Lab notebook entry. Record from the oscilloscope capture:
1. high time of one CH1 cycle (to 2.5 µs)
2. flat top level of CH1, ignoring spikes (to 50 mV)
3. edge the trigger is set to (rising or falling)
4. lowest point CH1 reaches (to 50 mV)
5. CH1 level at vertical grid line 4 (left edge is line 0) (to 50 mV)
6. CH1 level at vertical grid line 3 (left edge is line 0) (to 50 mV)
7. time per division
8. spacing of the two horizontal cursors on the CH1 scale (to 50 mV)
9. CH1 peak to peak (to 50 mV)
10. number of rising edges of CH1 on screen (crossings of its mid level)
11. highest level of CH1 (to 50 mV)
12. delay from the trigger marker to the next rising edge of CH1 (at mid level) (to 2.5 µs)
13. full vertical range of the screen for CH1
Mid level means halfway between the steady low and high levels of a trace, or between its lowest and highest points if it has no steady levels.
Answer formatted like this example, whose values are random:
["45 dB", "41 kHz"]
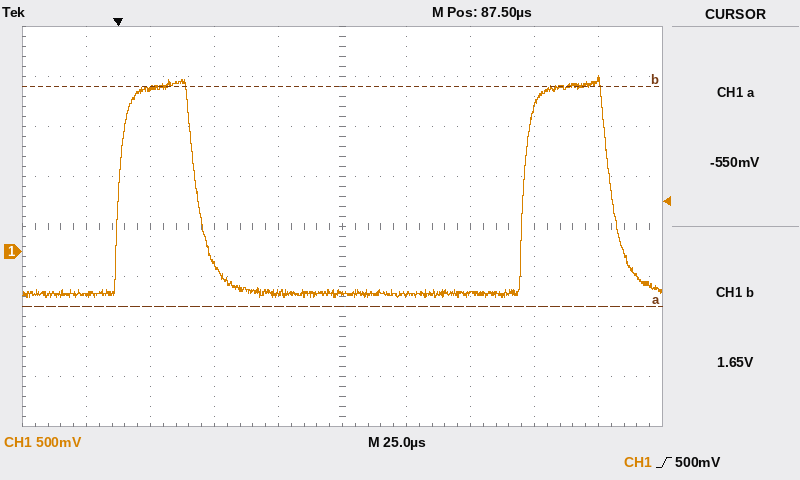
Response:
["32.5 µs", "1.65 V", "rising", "-450 mV", "-400 mV", "-150 mV", "25 µs", "2.20 V", "2.20 V", "2", "1.75 V", "157.5 µs", "4 V"]
